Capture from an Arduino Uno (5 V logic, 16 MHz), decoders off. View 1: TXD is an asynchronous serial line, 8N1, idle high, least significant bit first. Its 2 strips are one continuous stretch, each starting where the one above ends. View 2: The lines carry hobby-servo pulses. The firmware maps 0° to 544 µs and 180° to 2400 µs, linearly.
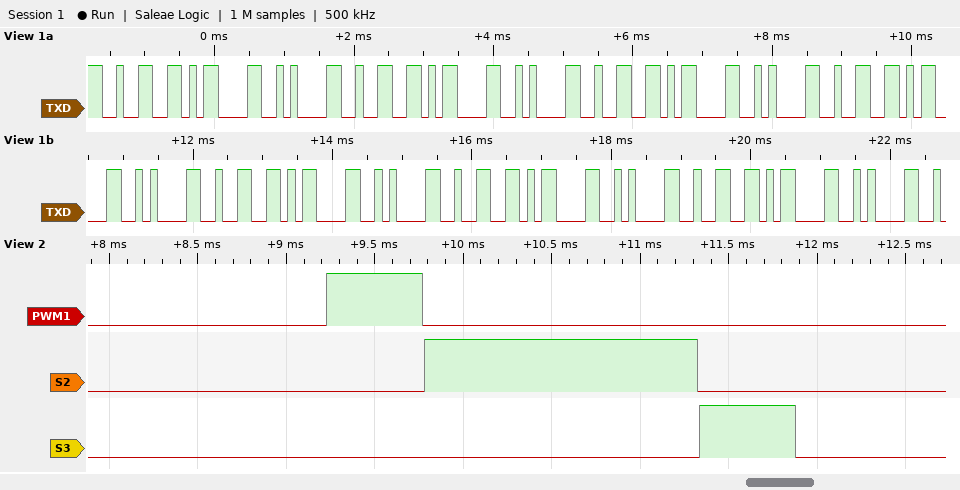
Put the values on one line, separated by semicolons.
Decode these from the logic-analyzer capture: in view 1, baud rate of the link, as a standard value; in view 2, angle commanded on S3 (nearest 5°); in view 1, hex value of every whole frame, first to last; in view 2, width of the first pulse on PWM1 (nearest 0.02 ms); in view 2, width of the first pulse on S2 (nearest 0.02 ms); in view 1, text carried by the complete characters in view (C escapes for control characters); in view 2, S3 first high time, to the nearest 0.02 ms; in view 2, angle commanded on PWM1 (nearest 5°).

9600 baud; 0°; 0x32 0x0D 0x0A 0x32 0x0D 0x0A 0x32 0x0D 0x0A 0x32 0x0D 0x0A 0x32 0x0D 0x0A 0x32 0x0D 0x0A 0x32 0x0D 0x0A; 0.54 ms; 1.54 ms; "2\r\n2\r\n2\r\n2\r\n2\r\n2\r\n2\r\n"; 0.54 ms; 0°
